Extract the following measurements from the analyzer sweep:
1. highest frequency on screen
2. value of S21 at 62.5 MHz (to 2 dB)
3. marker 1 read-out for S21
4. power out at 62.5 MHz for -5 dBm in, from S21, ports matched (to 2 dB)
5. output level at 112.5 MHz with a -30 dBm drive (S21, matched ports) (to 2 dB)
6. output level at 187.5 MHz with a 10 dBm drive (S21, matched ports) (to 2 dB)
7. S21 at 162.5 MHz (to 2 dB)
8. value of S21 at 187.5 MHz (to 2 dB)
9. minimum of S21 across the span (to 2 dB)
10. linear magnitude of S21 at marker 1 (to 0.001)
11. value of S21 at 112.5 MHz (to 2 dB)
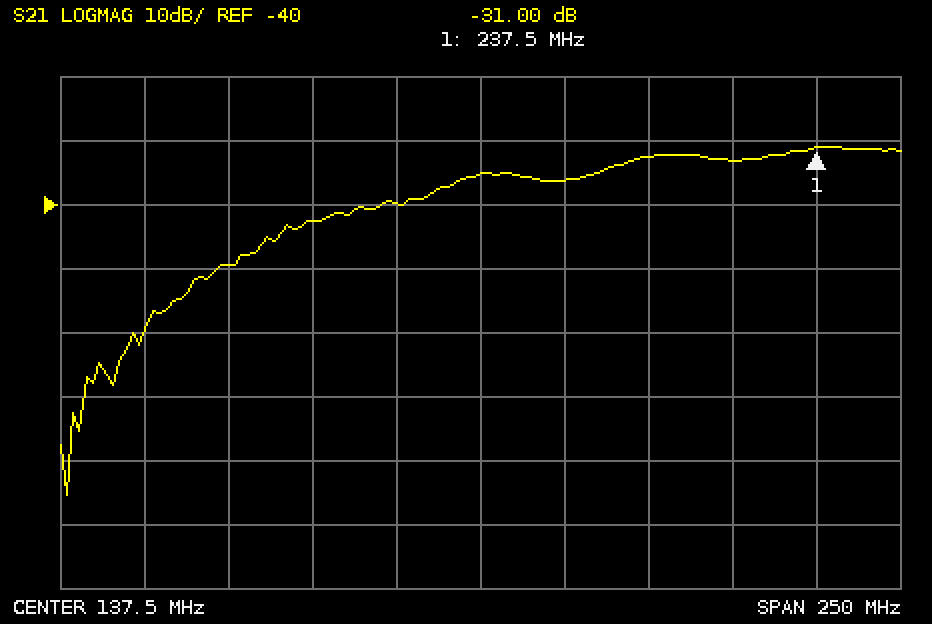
262.5 MHz
-50 dB
-31.00 dB
-54 dBm
-70 dBm
-22 dBm
-36 dB
-32 dB
-86 dB
0.028
-40 dB
